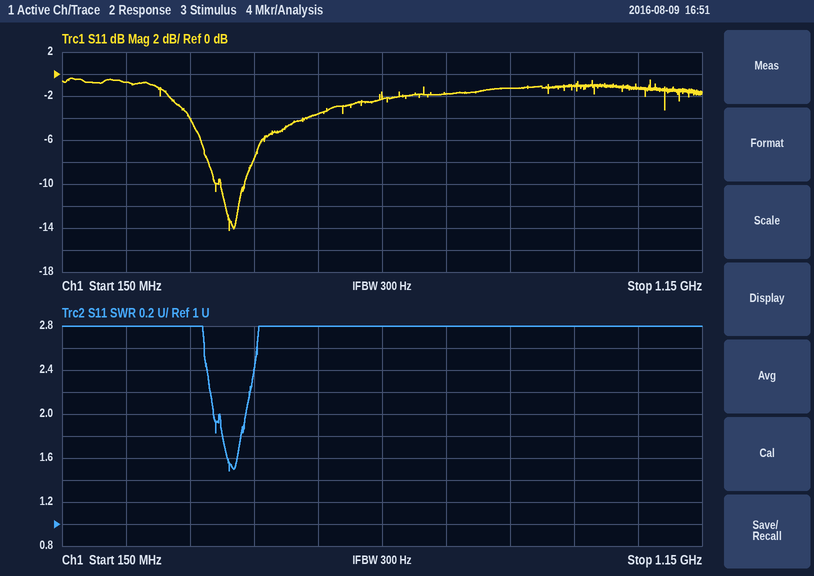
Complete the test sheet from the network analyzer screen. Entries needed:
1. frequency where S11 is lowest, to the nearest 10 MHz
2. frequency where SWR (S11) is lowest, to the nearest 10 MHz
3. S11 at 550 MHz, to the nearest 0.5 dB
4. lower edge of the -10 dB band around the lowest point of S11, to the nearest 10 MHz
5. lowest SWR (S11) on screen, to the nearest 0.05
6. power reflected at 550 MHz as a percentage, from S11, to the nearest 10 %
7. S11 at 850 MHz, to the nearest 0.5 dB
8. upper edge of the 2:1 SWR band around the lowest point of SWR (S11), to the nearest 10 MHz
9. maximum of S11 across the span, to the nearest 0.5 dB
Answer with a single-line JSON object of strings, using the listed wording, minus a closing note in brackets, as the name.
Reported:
{"frequency where S11 is lowest, to the nearest 10 MHz": "410 MHz", "frequency where SWR (S11) is lowest, to the nearest 10 MHz": "410 MHz", "S11 at 550 MHz, to the nearest 0.5 dB": "-3.5 dB", "lower edge of the -10 dB band around the lowest point of S11, to the nearest 10 MHz": "400 MHz", "lowest SWR (S11) on screen, to the nearest 0.05": "1.50", "power reflected at 550 MHz as a percentage, from S11, to the nearest 10 %": "40 %", "S11 at 850 MHz, to the nearest 0.5 dB": "-1.5 dB", "upper edge of the 2:1 SWR band around the lowest point of SWR (S11), to the nearest 10 MHz": "440 MHz", "maximum of S11 across the span, to the nearest 0.5 dB": "-0.5 dB"}
